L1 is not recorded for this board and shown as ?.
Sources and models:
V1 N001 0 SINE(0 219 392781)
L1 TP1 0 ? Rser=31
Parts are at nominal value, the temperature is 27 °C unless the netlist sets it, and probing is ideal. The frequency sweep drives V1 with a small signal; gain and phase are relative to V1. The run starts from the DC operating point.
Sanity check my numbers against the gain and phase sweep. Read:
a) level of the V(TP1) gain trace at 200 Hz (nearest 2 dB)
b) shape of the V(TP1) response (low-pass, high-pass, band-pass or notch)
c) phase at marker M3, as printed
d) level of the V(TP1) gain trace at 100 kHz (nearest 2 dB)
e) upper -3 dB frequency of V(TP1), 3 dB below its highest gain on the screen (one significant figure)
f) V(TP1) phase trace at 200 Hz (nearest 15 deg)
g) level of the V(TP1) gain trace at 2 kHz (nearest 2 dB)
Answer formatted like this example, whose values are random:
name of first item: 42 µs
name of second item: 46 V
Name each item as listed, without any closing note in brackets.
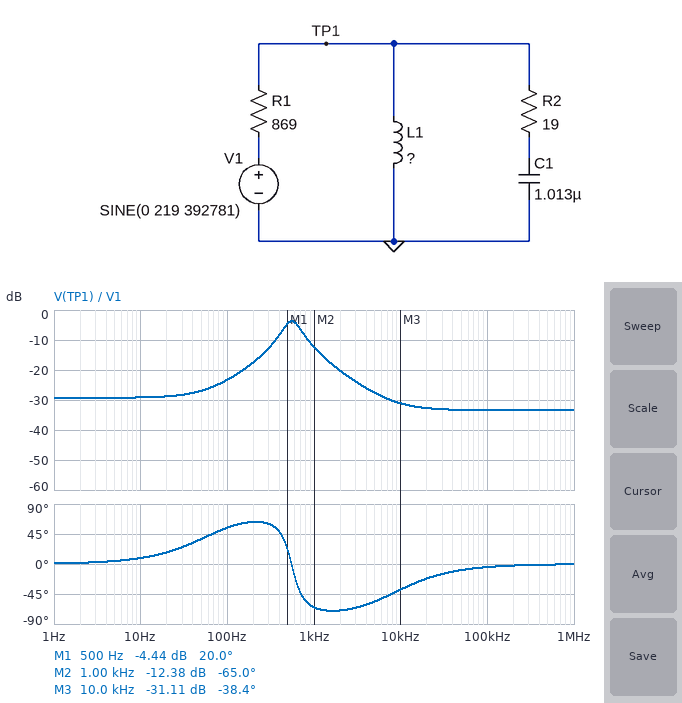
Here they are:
level of the V(TP1) gain trace at 200 Hz: -18 dB
shape of the V(TP1) response: band-pass
phase at marker M3, as printed: -38.4 deg
level of the V(TP1) gain trace at 100 kHz: -34 dB
upper -3 dB frequency of V(TP1), 3 dB below its highest gain on the screen: 700 Hz
V(TP1) phase trace at 200 Hz: 60 deg
level of the V(TP1) gain trace at 2 kHz: -20 dB
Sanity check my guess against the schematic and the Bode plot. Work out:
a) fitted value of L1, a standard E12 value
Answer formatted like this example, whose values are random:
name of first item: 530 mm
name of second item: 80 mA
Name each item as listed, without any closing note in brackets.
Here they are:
fitted value of L1, a standard E12 value: 82 mH
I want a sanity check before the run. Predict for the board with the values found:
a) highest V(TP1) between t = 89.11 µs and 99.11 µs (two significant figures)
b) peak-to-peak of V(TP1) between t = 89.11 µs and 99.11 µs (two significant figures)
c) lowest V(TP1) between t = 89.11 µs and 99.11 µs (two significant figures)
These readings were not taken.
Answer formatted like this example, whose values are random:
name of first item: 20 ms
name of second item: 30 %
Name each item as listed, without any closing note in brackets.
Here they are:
highest V(TP1) between t = 89.11 µs and 99.11 µs: 4.8 V
peak-to-peak of V(TP1) between t = 89.11 µs and 99.11 µs: 9.4 V
lowest V(TP1) between t = 89.11 µs and 99.11 µs: -4.6 V
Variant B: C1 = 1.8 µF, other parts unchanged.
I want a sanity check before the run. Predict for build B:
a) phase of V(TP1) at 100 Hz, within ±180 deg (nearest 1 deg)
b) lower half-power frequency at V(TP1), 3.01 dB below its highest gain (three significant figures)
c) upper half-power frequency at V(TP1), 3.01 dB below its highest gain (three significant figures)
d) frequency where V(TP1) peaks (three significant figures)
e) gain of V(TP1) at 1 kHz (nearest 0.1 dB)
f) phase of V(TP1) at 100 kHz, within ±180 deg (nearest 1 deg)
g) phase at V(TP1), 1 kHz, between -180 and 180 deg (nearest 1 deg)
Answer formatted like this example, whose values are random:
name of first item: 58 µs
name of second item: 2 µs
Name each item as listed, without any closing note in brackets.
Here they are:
phase of V(TP1) at 100 Hz, within ±180 deg: 53 deg
lower half-power frequency at V(TP1), 3.01 dB below its highest gain: 330 Hz
upper half-power frequency at V(TP1), 3.01 dB below its highest gain: 526 Hz
frequency where V(TP1) peaks: 417 Hz
gain of V(TP1) at 1 kHz: -18.4 dB
phase of V(TP1) at 100 kHz, within ±180 deg: -3 deg
phase at V(TP1), 1 kHz, between -180 and 180 deg: -68 deg
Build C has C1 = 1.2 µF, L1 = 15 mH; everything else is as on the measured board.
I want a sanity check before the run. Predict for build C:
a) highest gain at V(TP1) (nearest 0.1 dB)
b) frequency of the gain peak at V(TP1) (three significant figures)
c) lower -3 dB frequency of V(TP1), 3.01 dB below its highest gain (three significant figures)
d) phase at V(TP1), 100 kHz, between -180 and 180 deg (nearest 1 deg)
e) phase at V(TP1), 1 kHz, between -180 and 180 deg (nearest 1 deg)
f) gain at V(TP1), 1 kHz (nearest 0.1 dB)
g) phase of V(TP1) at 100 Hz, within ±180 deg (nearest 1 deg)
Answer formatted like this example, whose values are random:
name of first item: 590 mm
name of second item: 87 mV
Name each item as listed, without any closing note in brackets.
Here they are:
highest gain at V(TP1): -12.7 dB
frequency of the gain peak at V(TP1): 1.19 kHz
lower -3 dB frequency of V(TP1), 3.01 dB below its highest gain: 893 Hz
phase at V(TP1), 100 kHz, between -180 and 180 deg: -4 deg
phase at V(TP1), 1 kHz, between -180 and 180 deg: 22 deg
gain at V(TP1), 1 kHz: -14.0 dB
phase of V(TP1) at 100 Hz, within ±180 deg: 15 deg
